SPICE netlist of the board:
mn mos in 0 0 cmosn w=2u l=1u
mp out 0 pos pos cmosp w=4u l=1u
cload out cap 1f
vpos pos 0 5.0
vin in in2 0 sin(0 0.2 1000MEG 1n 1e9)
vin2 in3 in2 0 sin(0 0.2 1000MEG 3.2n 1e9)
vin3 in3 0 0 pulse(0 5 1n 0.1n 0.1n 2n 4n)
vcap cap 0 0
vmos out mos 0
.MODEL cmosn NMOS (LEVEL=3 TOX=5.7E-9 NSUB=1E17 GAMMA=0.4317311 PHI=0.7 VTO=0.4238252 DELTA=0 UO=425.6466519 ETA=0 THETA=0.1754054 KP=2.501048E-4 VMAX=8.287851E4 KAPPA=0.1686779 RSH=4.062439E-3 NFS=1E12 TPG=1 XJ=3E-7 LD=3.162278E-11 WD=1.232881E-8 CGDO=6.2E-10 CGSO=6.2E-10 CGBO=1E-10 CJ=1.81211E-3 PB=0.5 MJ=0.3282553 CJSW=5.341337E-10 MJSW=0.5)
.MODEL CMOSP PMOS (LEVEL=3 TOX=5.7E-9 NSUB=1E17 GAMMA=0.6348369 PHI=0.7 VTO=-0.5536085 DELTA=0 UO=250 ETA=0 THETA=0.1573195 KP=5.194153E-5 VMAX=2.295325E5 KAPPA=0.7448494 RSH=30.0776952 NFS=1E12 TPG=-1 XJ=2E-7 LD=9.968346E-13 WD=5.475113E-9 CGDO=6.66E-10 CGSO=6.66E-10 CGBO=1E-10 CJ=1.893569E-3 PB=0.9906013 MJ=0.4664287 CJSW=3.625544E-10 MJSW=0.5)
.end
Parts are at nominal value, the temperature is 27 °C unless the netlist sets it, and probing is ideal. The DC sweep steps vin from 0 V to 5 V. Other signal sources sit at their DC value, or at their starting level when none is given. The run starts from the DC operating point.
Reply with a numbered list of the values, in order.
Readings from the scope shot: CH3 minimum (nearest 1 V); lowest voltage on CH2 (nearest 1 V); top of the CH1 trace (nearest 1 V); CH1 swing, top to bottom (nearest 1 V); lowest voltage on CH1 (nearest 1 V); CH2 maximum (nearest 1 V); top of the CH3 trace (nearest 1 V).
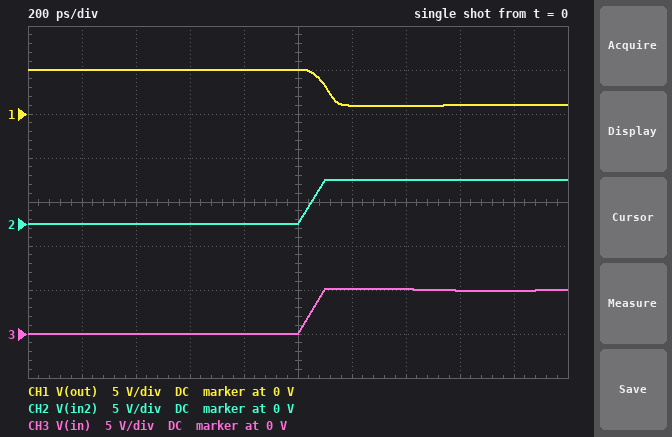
1. 0 V
2. 0 V
3. 5 V
4. 4 V
5. 1 V
6. 5 V
7. 5 V
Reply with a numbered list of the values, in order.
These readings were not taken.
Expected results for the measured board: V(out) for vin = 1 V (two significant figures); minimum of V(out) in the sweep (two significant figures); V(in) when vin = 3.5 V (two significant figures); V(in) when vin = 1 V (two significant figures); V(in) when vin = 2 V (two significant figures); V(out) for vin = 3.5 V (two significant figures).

1. 4.9 V
2. 970 mV
3. 3.5 V
4. 1.0 V
5. 2.0 V
6. 2.5 V
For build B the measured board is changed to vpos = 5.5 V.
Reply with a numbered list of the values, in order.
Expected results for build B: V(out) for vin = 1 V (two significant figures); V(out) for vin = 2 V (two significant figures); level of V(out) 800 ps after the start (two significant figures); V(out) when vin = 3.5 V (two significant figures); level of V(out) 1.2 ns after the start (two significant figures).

1. 5.4 V
2. 4.9 V
3. 5.5 V
4. 3.4 V
5. 1.2 V
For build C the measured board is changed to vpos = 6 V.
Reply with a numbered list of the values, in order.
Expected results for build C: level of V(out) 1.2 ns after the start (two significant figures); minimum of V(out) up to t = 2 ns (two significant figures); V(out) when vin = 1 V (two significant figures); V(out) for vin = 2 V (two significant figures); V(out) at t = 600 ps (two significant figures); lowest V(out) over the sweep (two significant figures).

1. 1.7 V
2. 1.5 V
3. 5.9 V
4. 5.4 V
5. 6.0 V
6. 1.6 V
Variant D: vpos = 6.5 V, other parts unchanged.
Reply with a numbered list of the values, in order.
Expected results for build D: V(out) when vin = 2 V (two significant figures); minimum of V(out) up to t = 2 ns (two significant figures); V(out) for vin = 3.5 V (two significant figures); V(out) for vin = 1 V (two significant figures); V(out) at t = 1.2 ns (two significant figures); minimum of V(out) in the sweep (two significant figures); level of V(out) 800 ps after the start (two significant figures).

1. 5.9 V
2. 2.1 V
3. 4.8 V
4. 6.4 V
5. 2.8 V
6. 2.3 V
7. 6.5 V
